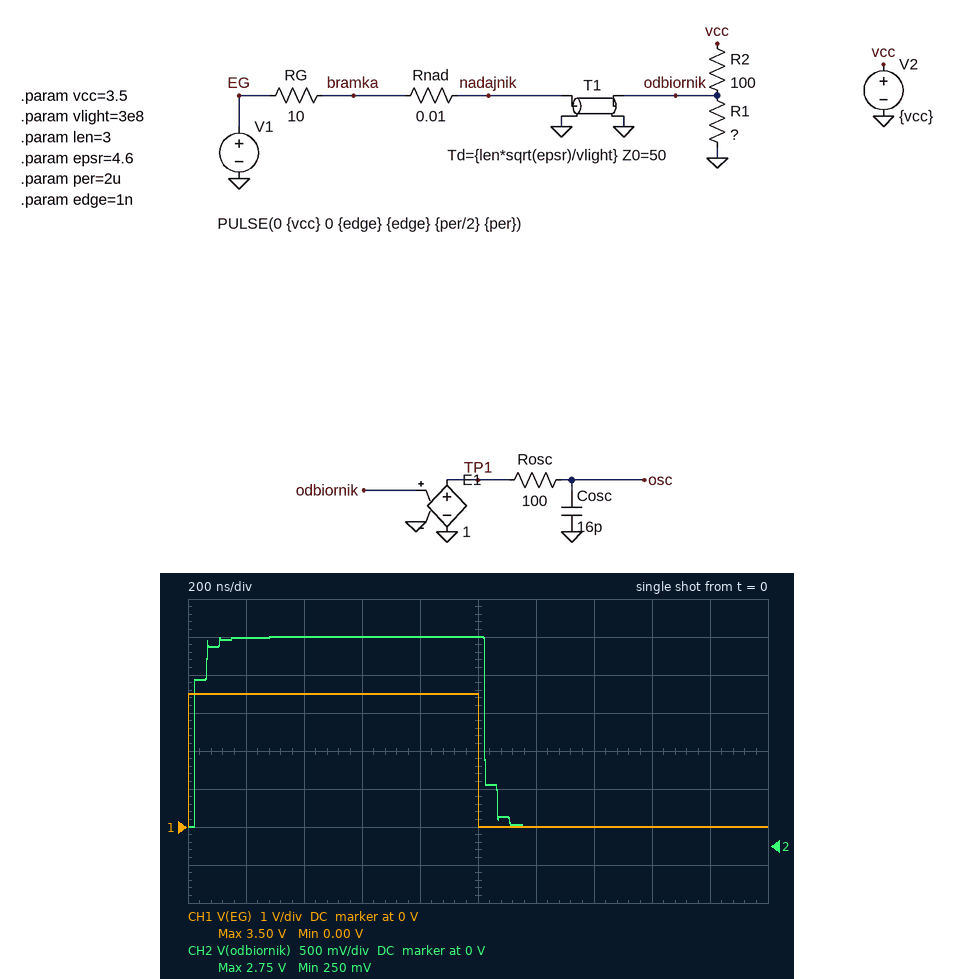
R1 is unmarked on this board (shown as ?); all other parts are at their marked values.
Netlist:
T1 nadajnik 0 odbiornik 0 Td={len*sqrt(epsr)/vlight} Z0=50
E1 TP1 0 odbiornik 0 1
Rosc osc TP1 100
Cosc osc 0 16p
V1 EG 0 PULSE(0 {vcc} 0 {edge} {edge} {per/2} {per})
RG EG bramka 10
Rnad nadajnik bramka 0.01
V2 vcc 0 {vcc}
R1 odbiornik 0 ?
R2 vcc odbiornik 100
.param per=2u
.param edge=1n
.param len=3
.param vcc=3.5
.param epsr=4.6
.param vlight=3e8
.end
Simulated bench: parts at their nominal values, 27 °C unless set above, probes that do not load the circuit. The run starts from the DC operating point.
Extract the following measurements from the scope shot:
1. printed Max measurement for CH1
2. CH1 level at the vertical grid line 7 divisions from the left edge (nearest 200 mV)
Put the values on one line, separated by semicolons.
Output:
3.50 V; 0 V
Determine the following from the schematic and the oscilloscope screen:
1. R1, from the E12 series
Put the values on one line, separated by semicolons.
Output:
33 Ω
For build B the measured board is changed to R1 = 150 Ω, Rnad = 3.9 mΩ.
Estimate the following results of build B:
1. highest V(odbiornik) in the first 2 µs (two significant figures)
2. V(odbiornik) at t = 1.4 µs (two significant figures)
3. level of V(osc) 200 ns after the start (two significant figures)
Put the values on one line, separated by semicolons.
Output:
3.5 V; 300 mV; 3.3 V
